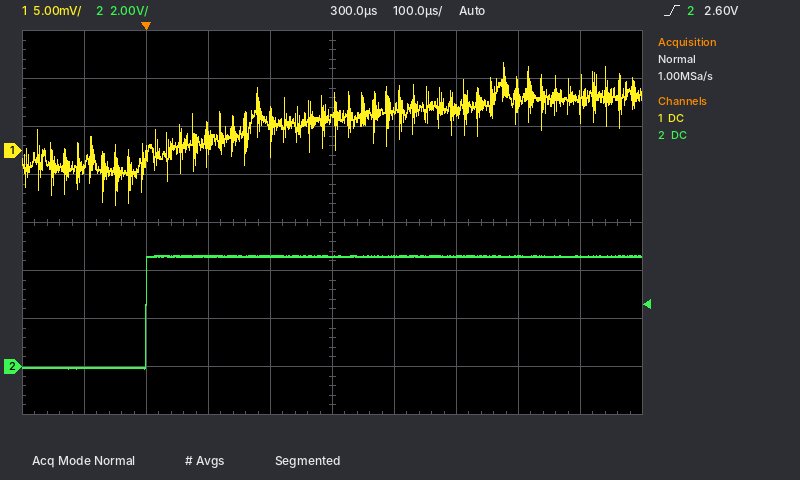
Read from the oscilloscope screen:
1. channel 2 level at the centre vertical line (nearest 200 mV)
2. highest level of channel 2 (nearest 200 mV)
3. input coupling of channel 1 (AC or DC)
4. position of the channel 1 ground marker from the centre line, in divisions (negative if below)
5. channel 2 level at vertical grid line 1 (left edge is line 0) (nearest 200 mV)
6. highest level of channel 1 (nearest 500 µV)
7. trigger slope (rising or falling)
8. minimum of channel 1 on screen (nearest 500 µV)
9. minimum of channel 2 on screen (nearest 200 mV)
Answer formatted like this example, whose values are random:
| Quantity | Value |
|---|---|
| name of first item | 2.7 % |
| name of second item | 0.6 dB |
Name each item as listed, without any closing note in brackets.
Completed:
| Quantity | Value |
|---|---|
| channel 2 level at the centre vertical line | 4.6 V |
| highest level of channel 2 | 4.6 V |
| input coupling of channel 1 | DC |
| position of the channel 1 ground marker from the centre line, in divisions | +1.5 div |
| channel 2 level at vertical grid line 1 (left edge is line 0) | 0.0 V |
| highest level of channel 1 | 9.0 mV |
| trigger slope | rising |
| minimum of channel 1 on screen | -5.5 mV |
| minimum of channel 2 on screen | 0.0 V |
